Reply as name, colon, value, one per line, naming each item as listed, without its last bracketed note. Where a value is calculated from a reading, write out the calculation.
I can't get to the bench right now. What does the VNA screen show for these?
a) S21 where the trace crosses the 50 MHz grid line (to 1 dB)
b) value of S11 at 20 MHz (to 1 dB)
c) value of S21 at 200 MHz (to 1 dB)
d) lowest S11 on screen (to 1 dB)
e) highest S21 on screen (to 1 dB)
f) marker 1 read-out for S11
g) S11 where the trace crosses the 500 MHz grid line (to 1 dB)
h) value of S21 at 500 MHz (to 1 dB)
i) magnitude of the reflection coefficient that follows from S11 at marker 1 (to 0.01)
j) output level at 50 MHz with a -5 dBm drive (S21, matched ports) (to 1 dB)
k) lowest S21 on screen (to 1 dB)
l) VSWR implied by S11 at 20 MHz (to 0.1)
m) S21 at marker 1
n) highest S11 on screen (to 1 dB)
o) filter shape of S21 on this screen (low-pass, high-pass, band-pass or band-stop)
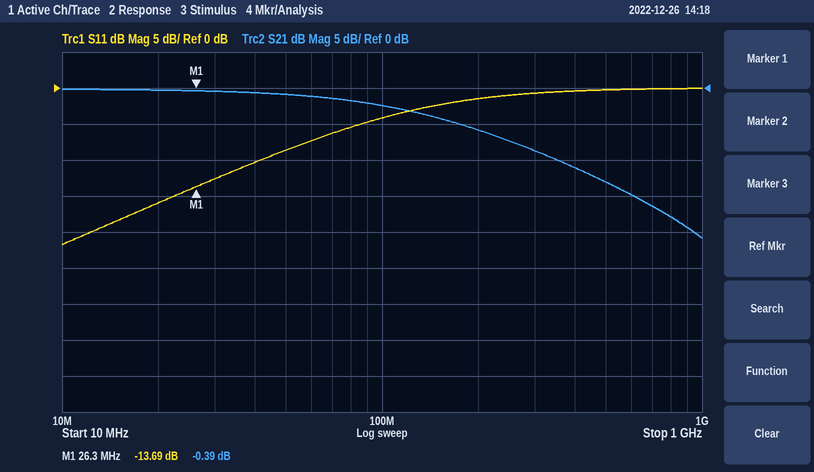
S21 where the trace crosses the 50 MHz grid line: -1 dB
value of S11 at 20 MHz: -16 dB
value of S21 at 200 MHz: -6 dB
lowest S11 on screen: -22 dB
highest S21 on screen: 0 dB
marker 1 read-out for S11: -13.69 dB
S11 where the trace crosses the 500 MHz grid line: 0 dB
value of S21 at 500 MHz: -13 dB
magnitude of the reflection coefficient that follows from S11 at marker 1: 10^(-13.69/20) ≈ 0.21
output level at 50 MHz with a -5 dBm drive (S21, matched ports): -5 dBm + (-1 dB) = -6 dBm
lowest S21 on screen: -21 dB
VSWR implied by S11 at 20 MHz: |Γ| = 10^(-16/20) = 0.1585; VSWR = (1 + 0.1585)/(1 − 0.1585) ≈ 1.4
S21 at marker 1: -0.39 dB
highest S11 on screen: 0 dB
filter shape of S21 on this screen: low-pass
